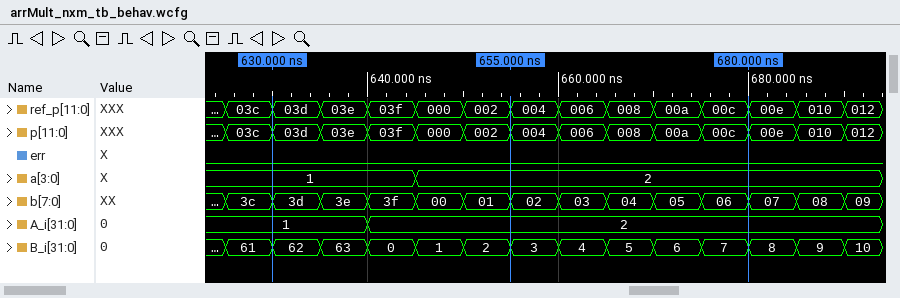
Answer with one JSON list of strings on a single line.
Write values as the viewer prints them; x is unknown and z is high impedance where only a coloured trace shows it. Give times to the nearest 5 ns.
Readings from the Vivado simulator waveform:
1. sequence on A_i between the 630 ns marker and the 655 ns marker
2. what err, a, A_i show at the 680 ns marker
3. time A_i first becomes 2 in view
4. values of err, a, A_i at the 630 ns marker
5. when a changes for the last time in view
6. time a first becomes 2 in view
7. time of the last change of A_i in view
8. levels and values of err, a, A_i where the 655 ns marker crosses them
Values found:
["1, 2", "err=0, a=2, A_i=2", "640 ns", "err=0, a=1, A_i=1", "645 ns", "645 ns", "640 ns", "err=0, a=2, A_i=2"]
